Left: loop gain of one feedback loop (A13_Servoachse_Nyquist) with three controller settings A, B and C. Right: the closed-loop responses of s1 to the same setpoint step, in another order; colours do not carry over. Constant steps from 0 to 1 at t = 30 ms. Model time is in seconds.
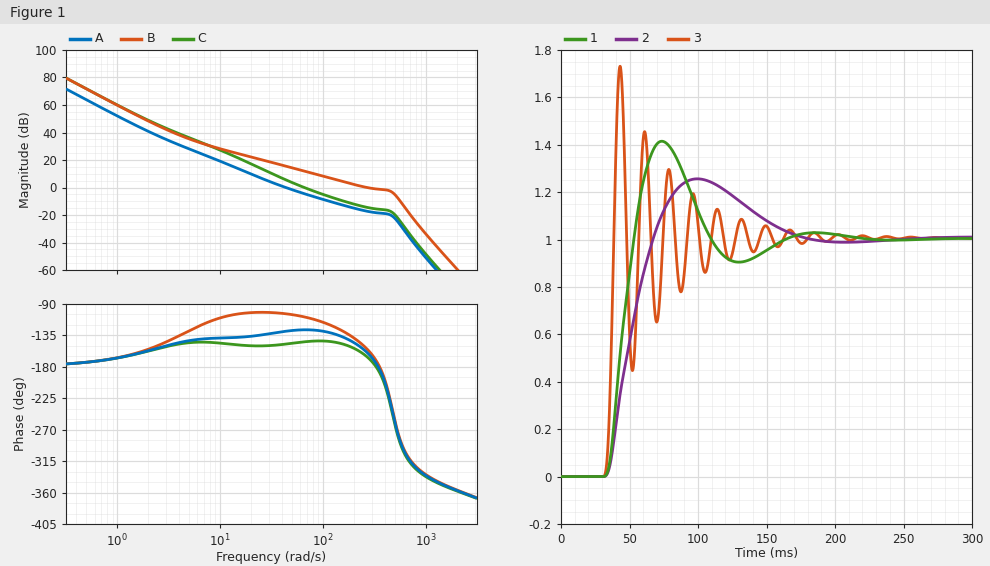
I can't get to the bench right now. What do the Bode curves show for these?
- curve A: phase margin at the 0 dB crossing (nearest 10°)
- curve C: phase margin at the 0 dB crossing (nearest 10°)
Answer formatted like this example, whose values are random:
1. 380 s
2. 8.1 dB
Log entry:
1. 50°
2. 40°
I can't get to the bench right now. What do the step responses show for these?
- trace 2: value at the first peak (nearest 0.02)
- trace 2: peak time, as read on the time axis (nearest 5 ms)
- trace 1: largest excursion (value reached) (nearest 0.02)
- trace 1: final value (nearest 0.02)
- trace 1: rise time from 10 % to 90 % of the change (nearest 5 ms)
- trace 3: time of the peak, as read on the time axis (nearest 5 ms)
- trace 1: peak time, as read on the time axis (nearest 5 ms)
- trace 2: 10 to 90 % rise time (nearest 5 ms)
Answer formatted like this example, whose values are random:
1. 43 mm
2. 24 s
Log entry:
1. 1.26
2. 100 ms
3. 1.42
4. 1.00
5. 15 ms
6. 45 ms
7. 75 ms
8. 25 ms
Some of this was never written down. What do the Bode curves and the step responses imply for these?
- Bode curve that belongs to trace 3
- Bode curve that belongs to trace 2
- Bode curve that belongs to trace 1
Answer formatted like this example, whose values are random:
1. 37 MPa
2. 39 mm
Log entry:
1. B
2. A
3. C
